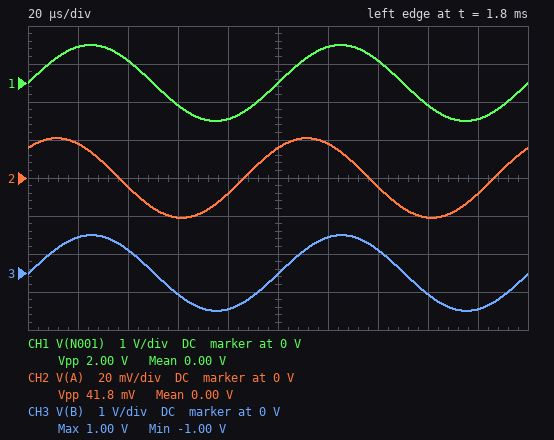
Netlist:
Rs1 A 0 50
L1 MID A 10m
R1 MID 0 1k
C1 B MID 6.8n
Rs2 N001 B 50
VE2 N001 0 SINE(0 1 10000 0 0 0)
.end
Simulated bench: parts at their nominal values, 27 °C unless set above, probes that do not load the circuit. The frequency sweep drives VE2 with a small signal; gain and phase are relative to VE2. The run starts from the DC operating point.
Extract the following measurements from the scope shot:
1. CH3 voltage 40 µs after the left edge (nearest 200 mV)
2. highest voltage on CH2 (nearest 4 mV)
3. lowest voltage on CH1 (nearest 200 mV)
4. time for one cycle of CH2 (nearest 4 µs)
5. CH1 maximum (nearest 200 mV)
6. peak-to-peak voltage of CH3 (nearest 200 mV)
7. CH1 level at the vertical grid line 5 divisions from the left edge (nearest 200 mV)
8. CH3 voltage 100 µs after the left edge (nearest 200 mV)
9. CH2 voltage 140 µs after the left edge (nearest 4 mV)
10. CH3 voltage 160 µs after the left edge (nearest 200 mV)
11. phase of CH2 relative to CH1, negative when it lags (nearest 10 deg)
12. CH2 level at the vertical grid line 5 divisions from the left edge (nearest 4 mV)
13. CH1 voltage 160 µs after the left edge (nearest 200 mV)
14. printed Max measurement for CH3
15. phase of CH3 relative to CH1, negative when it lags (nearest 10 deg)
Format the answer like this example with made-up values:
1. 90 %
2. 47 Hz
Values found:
1. 600 mV
2. 20 mV
3. -1.0 V
4. 100 µs
5. 1.0 V
6. 2.0 V
7. 0 V
8. 0 V
9. -4 mV
10. -600 mV
11. 50 deg
12. 16 mV
13. -600 mV
14. 1.00 V
15. 0 deg
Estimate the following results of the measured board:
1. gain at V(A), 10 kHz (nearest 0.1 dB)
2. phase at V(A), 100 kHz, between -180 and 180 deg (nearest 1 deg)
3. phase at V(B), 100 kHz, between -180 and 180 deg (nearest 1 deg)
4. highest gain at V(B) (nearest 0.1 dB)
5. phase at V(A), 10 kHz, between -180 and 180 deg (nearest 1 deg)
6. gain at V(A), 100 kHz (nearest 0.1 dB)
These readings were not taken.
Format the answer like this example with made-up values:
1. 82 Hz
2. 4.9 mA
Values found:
1. -33.6 dB
2. -76 deg
3. 0 deg
4. 0 dB
5. 49 deg
6. -42.3 dB
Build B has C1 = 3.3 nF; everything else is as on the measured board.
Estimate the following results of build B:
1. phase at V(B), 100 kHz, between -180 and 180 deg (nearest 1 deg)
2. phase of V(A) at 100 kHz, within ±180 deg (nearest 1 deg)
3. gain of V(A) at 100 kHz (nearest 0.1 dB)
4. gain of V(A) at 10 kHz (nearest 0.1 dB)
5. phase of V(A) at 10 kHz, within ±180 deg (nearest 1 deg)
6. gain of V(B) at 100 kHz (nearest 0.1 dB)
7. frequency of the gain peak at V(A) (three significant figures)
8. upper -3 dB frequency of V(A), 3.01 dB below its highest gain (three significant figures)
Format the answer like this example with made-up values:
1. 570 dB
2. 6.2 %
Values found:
1. -1 deg
2. -63 deg
3. -42.7 dB
4. -40.7 dB
5. 55 deg
6. -0.4 dB
7. 27.7 kHz
8. 60.2 kHz
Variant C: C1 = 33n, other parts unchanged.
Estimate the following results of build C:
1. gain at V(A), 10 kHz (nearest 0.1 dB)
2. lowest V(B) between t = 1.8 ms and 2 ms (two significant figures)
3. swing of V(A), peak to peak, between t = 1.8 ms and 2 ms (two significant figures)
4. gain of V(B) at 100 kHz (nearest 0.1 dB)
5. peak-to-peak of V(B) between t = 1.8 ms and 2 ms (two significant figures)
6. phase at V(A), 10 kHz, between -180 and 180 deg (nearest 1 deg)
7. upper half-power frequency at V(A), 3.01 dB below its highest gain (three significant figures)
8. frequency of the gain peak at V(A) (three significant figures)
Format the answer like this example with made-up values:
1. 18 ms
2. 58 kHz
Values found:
1. -18.8 dB
2. -860 mV
3. 230 mV
4. -0.4 dB
5. 1.7 V
6. -21 deg
7. 12.4 kHz
8. 8.76 kHz
